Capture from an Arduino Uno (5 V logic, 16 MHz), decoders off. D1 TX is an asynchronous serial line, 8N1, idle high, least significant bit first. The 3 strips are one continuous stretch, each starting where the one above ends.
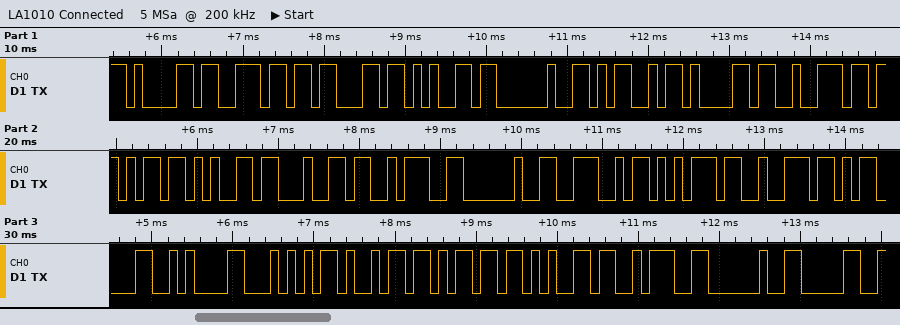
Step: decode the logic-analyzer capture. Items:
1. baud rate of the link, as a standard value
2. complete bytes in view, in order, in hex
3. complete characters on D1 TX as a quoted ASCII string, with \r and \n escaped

9600 baud
61 6E 63 65 20 4D 61 72 6B 65 64 3A 20 4E 75 72 0D 0A 54 69 6D 65 3A 20 30
"ance Marked: Nur\r\nTime: 0"
